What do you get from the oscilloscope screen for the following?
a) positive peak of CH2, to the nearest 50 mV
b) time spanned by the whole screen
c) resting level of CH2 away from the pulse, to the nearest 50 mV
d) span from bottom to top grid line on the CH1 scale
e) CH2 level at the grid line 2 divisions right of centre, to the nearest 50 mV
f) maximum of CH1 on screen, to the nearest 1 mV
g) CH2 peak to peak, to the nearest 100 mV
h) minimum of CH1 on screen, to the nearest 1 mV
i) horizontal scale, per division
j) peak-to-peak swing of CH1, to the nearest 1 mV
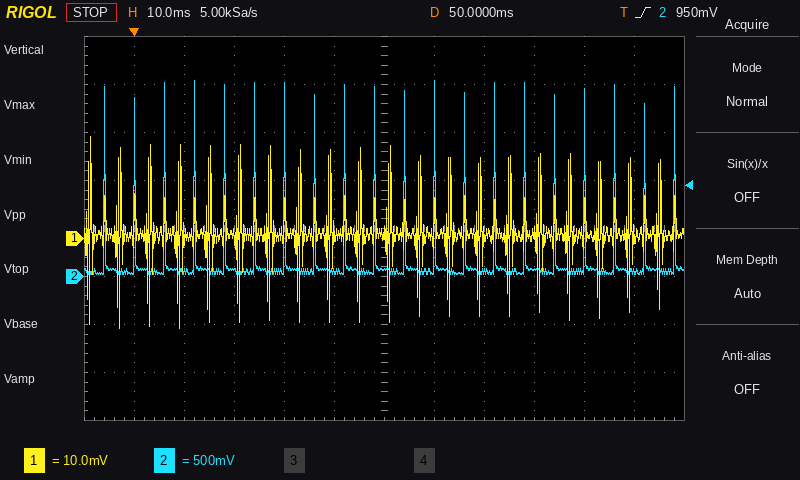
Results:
2.05 V
120 ms
50 mV
80 mV
50 mV
21 mV
2.00 V
-19 mV
10 ms
40 mV
